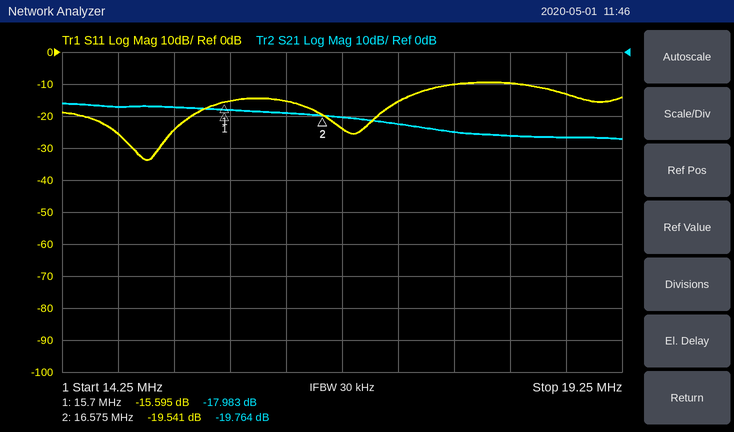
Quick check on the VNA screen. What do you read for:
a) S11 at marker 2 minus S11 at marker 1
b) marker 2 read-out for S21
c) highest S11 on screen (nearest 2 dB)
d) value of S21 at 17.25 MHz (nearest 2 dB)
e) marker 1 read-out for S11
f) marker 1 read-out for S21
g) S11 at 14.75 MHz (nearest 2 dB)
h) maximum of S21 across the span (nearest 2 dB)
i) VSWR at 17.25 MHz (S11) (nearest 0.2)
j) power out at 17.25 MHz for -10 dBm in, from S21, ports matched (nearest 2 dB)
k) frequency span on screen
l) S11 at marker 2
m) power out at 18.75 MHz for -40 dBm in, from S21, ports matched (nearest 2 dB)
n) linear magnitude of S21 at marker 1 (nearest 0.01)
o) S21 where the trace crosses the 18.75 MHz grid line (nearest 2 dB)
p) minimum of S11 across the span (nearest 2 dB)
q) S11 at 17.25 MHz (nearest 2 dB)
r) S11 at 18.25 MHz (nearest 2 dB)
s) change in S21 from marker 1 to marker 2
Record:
-3.946 dB
-19.764 dB
-10 dB
-22 dB
-15.595 dB
-17.983 dB
-26 dB
-16 dB
1.4
-32 dBm
5 MHz
-19.541 dB
-66 dBm
0.13
-26 dB
-34 dB
-16 dB
-10 dB
-1.781 dB
